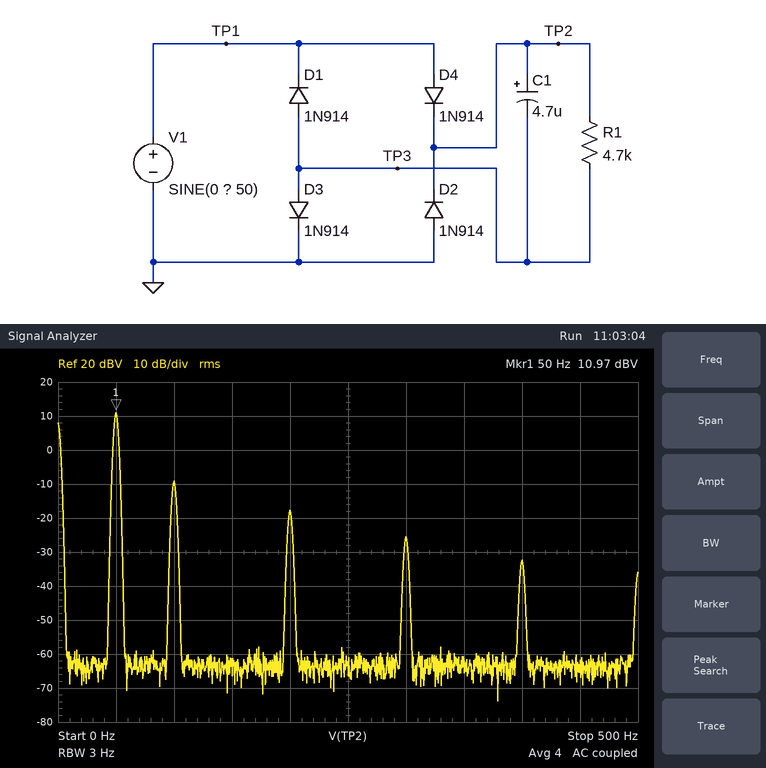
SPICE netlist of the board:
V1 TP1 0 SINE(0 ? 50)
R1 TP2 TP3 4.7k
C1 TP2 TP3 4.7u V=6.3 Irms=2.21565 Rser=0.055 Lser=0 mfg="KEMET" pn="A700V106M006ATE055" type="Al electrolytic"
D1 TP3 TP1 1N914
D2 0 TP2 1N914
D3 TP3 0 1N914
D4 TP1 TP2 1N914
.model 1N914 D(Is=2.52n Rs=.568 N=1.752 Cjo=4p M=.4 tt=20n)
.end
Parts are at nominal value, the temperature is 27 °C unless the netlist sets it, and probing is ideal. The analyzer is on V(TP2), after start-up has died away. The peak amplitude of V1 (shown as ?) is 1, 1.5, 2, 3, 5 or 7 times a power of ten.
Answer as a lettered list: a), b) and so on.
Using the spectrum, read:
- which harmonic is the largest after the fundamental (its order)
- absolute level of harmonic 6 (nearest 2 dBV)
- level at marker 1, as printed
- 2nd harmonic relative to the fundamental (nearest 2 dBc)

a) 2
b) -26 dBV
c) 10.97 dBV
d) -20 dBc
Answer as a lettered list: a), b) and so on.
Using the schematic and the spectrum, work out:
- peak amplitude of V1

a) 10 V
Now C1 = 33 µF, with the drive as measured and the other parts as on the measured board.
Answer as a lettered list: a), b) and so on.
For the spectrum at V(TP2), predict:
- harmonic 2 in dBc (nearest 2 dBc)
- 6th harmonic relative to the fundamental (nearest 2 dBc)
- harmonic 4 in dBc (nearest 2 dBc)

a) -36 dBc
b) -46 dBc
c) -42 dBc
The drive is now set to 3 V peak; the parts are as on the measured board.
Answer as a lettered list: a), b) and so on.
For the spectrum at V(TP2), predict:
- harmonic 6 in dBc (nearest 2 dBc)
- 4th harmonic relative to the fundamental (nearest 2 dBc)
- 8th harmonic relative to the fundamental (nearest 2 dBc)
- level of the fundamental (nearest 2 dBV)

a) -40 dBc
b) -32 dBc
c) -46 dBc
d) 0 dBV
